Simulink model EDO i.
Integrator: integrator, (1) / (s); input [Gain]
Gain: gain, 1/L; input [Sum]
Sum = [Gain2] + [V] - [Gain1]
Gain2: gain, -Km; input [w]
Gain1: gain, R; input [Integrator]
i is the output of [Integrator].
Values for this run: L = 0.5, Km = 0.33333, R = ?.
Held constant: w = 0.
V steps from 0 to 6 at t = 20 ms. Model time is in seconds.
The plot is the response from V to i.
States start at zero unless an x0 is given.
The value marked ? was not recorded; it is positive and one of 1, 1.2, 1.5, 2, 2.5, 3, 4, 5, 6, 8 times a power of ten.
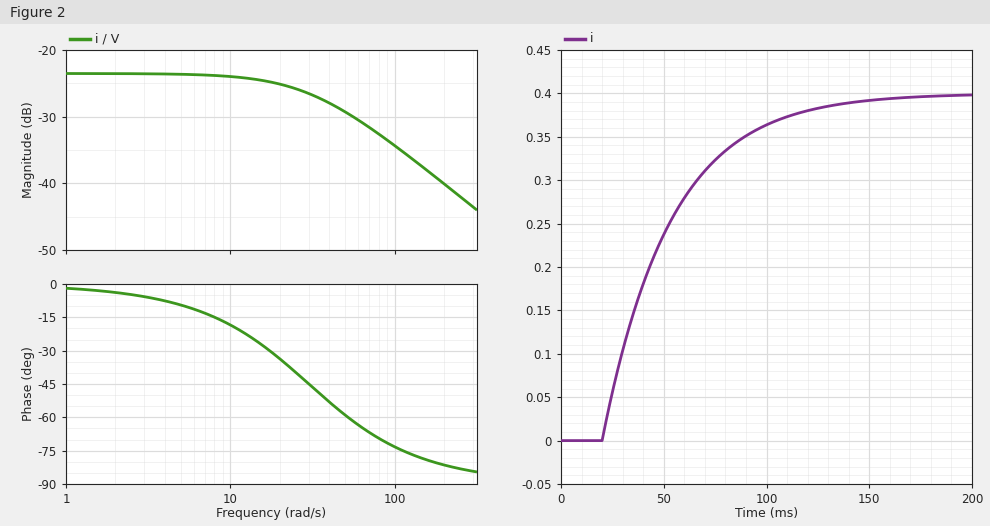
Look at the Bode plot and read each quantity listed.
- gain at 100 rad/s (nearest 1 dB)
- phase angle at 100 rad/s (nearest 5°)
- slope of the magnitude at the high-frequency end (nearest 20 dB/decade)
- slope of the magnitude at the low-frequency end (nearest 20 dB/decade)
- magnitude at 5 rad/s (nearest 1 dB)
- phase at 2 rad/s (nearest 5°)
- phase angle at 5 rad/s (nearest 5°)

-34 dB
-75°
-20 dB/decade
0 dB/decade
-24 dB
-5°
-10°
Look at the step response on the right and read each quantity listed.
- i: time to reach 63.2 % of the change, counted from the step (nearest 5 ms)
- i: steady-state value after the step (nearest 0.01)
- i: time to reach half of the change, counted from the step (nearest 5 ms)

35 ms
0.40
25 ms
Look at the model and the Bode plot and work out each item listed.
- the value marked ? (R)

15
